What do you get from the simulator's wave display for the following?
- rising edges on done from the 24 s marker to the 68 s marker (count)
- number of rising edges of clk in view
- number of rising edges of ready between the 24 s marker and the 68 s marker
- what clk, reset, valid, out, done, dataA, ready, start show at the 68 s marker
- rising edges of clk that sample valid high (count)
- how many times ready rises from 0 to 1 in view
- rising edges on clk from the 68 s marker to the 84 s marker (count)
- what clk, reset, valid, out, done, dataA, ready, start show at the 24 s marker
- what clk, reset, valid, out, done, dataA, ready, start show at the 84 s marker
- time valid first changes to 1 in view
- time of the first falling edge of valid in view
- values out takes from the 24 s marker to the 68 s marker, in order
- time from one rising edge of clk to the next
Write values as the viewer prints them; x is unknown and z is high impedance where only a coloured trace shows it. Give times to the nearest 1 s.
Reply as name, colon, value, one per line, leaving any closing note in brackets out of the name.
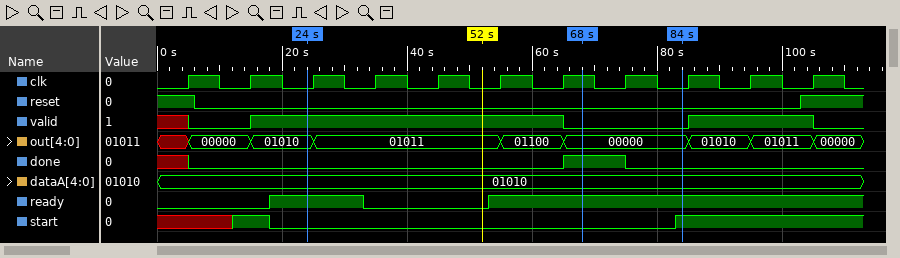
rising edges on done from the 24 s marker to the 68 s marker: 1
number of rising edges of clk in view: 11
number of rising edges of ready between the 24 s marker and the 68 s marker: 1
what clk, reset, valid, out, done, dataA, ready, start show at the 68 s marker: clk=1, reset=0, valid=0, out=00000, done=1, dataA=01010, ready=1, start=0
rising edges of clk that sample valid high: 7
how many times ready rises from 0 to 1 in view: 2
rising edges on clk from the 68 s marker to the 84 s marker: 1
what clk, reset, valid, out, done, dataA, ready, start show at the 24 s marker: clk=0, reset=0, valid=1, out=01010, done=0, dataA=01010, ready=1, start=0
what clk, reset, valid, out, done, dataA, ready, start show at the 84 s marker: clk=0, reset=0, valid=0, out=00000, done=0, dataA=01010, ready=1, start=1
time valid first changes to 1 in view: 15 s
time of the first falling edge of valid in view: 65 s
values out takes from the 24 s marker to the 68 s marker, in order: 01010, 01011, 01100, 00000
time from one rising edge of clk to the next: 10 s
